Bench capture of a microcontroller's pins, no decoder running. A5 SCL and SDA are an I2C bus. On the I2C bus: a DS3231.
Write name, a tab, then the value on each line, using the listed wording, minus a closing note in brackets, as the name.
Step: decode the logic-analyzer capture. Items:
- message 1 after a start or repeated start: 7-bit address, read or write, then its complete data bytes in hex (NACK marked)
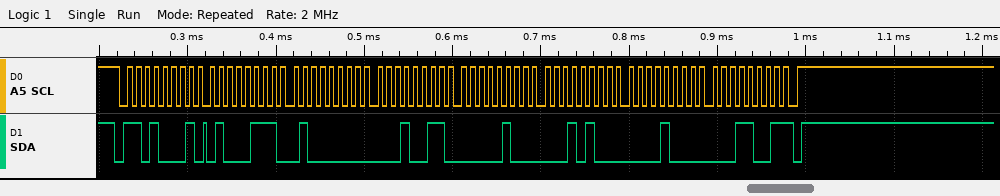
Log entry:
message 1 after a start or repeated start: 7-bit address, read or write, then its complete data bytes in hex	0x68 read: 47 40 13 04 14 08 19 NACK
